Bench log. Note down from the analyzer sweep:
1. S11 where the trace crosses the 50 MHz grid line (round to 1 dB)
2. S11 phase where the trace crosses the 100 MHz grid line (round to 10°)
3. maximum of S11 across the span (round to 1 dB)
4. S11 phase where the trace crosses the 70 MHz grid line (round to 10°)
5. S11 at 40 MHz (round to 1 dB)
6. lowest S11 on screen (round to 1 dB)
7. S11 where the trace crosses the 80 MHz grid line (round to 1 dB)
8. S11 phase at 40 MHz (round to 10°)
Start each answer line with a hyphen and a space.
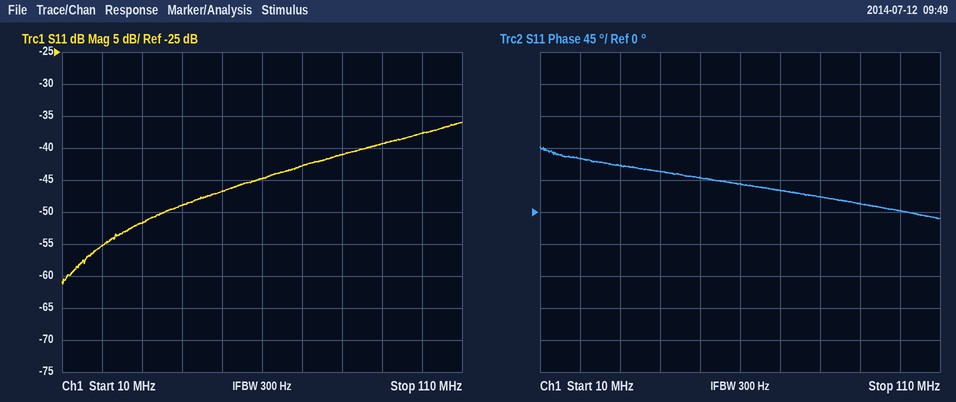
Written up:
- -47 dB
- 0°
- -36 dB
- 30°
- -49 dB
- -61 dB
- -41 dB
- 60°
